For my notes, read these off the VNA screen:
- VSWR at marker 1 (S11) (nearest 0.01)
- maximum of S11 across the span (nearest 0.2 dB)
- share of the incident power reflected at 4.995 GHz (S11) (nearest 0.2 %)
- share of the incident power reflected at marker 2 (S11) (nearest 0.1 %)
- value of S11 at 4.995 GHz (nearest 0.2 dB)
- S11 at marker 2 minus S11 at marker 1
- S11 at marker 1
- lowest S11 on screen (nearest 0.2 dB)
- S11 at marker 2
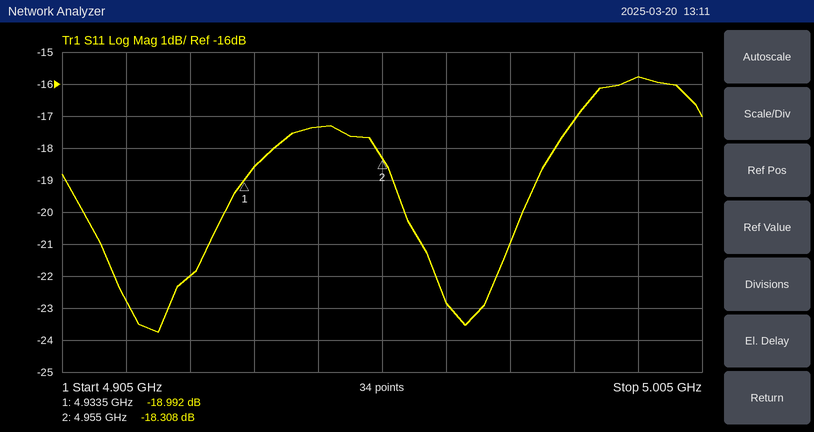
1.25
-15.8 dB
2.6 %
1.5 %
-15.8 dB
0.684 dB
-18.992 dB
-23.8 dB
-18.308 dB
